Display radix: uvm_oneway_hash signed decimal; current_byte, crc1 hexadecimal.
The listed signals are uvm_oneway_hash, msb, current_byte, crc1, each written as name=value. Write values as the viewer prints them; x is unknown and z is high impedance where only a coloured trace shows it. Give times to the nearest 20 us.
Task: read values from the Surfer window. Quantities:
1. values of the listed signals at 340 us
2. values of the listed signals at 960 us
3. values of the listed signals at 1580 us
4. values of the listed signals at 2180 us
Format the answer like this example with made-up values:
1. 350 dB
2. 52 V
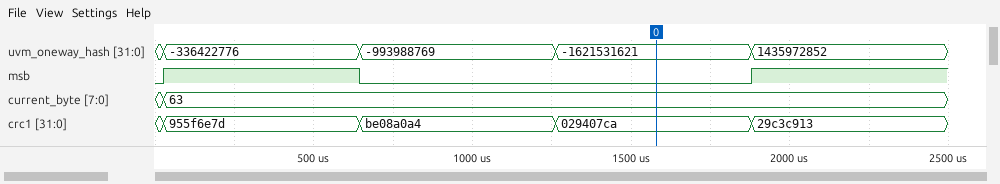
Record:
1. uvm_oneway_hash=-336422776, msb=1, current_byte=63, crc1=955f6e7d
2. uvm_oneway_hash=-993988769, msb=0, current_byte=63, crc1=be08a0a4
3. uvm_oneway_hash=-1621531621, msb=0, current_byte=63, crc1=029407ca
4. uvm_oneway_hash=1435972852, msb=1, current_byte=63, crc1=29c3c913
